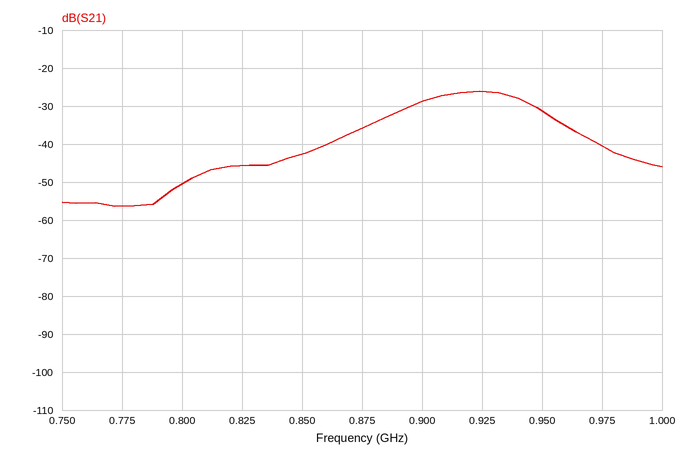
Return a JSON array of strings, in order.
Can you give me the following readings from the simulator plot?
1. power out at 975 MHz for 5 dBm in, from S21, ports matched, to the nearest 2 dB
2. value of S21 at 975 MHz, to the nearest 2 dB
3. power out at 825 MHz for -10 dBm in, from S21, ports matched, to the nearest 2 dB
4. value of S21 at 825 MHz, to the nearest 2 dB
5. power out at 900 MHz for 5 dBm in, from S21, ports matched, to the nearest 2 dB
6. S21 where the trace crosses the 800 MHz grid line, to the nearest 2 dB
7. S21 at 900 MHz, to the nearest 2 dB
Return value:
["-36 dBm", "-40 dB", "-56 dBm", "-46 dB", "-24 dBm", "-50 dB", "-28 dB"]
